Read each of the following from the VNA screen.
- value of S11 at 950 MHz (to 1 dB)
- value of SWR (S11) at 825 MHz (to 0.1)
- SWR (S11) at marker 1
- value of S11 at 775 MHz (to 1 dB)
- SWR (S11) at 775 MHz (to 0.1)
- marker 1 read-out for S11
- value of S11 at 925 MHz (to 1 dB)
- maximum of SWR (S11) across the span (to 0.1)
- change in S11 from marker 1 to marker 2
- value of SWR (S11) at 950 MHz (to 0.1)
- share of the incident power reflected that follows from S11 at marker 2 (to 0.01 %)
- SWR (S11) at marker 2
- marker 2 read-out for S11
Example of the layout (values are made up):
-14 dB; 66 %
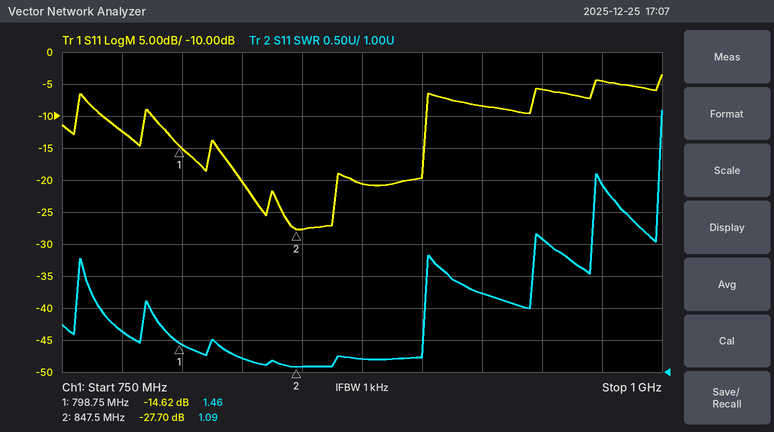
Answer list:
-6 dB; 1.2; 1.46; -12 dB; 1.6; -14.62 dB; -8 dB; 5.1; -13.08 dB; 3.1; 0.17 %; 1.09; -27.70 dB
